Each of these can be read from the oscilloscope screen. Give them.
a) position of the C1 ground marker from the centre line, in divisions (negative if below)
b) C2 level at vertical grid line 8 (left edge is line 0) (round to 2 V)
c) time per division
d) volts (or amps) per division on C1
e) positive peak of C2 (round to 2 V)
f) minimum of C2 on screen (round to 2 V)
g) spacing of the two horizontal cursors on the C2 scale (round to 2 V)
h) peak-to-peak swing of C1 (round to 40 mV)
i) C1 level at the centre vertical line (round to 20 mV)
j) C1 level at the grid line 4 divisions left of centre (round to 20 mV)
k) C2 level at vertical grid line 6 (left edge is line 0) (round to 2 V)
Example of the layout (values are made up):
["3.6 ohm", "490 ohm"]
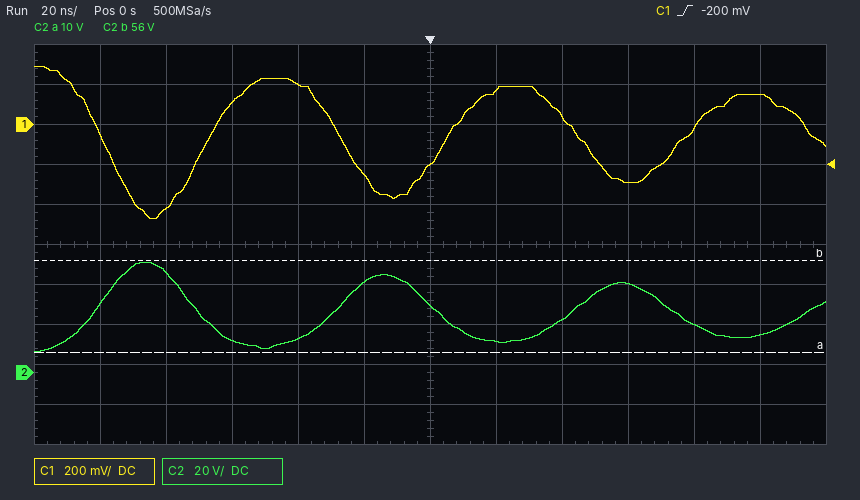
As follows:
["+3.0 div", "26 V", "20 ns", "200 mV", "56 V", "10 V", "46 V", "760 mV", "-200 mV", "-420 mV", "34 V"]
